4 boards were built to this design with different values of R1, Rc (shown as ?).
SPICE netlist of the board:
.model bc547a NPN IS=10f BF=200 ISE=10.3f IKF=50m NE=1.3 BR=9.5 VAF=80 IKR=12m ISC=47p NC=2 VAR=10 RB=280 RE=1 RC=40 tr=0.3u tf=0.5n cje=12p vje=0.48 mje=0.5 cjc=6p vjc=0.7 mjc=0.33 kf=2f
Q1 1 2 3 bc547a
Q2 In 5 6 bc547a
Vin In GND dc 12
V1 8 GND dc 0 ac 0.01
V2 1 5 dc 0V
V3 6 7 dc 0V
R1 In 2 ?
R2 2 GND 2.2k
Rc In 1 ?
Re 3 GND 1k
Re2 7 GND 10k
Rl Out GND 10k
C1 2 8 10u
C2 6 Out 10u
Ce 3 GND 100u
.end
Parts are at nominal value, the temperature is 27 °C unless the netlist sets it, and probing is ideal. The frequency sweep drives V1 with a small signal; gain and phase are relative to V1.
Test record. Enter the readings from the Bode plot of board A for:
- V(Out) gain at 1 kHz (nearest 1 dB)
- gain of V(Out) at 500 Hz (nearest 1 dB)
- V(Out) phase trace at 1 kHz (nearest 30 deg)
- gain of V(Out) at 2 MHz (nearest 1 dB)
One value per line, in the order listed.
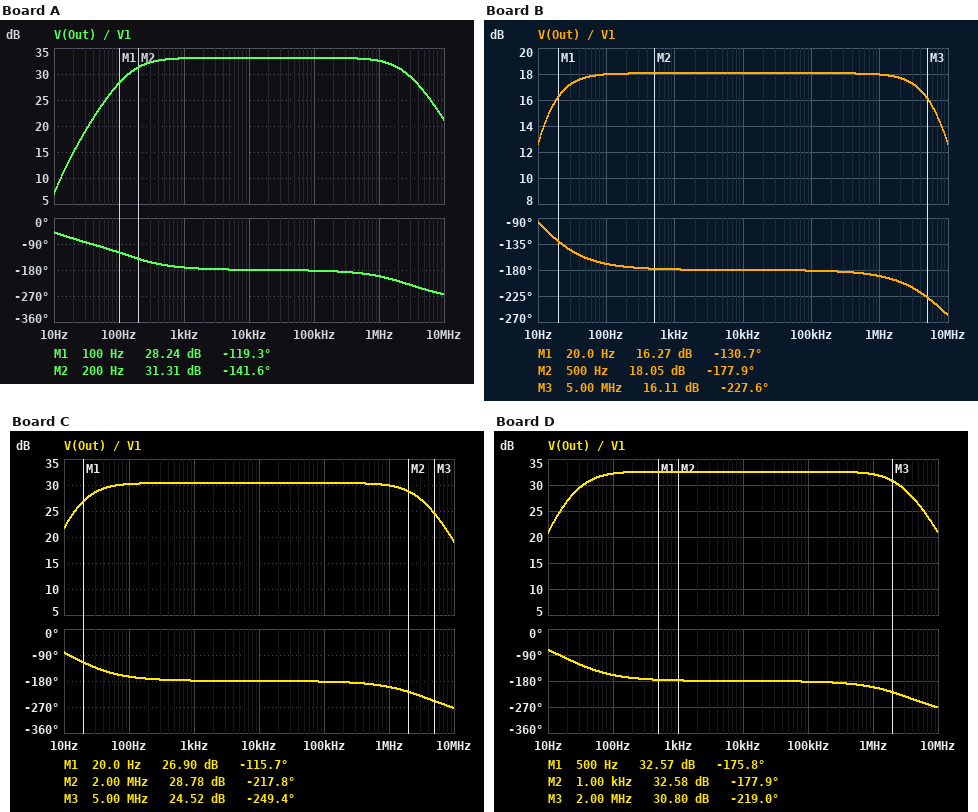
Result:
33 dB
33 dB
-180 deg
31 dB
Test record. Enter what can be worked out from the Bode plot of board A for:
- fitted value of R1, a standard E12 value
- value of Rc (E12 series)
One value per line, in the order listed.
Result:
4.7 kΩ
560 Ω
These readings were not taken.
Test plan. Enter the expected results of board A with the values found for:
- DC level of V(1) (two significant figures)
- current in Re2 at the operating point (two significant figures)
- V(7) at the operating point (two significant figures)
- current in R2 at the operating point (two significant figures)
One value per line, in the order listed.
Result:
10 V
960 µA
9.6 V
1.7 mA
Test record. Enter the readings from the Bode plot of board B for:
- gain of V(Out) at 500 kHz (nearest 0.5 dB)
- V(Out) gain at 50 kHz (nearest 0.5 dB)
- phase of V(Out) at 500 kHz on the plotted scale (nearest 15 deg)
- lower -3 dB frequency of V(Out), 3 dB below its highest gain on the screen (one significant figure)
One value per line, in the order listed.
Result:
18.0 dB
18.0 dB
-180 deg
10 Hz
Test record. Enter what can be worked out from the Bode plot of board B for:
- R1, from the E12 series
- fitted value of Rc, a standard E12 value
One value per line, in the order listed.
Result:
33 kΩ
1.5 kΩ
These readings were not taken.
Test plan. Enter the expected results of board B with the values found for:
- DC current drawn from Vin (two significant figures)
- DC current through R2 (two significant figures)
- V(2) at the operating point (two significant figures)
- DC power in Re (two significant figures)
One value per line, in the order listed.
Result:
1.6 mA
340 µA
750 mV
21 µW
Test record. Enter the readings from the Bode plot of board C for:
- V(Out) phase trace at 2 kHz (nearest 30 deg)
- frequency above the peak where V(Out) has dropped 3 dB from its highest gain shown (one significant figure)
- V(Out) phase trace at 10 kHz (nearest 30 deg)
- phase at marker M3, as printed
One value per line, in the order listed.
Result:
-180 deg
3 MHz
-180 deg
-249.4 deg
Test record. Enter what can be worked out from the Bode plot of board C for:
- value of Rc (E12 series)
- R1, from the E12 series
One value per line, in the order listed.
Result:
3.3 kΩ
27 kΩ
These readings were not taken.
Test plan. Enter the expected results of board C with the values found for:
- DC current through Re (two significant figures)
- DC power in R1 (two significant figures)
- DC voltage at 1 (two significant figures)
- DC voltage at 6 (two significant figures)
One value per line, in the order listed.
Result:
280 µA
4.6 mW
11 V
10 V
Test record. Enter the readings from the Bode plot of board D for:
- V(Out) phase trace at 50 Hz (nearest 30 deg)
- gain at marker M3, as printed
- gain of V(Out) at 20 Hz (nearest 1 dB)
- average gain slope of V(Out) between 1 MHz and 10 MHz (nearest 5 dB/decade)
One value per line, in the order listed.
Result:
-150 deg
30.80 dB
27 dB
-10 dB/decade
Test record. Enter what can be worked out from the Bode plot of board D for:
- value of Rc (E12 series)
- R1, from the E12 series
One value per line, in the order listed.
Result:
2.7 kΩ
22 kΩ
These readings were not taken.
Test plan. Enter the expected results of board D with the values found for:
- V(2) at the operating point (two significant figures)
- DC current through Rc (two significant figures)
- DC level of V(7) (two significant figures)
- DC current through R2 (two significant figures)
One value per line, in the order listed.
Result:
1.1 V
450 µA
10 V
490 µA
